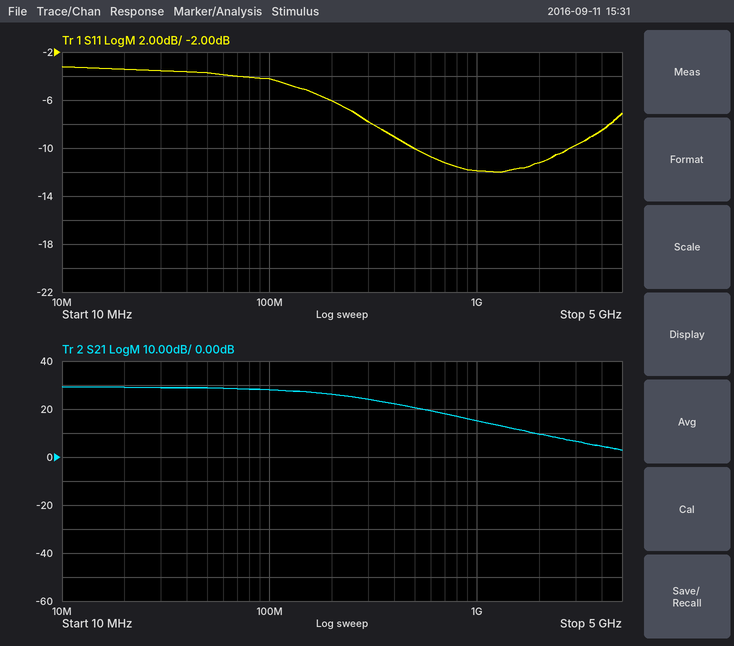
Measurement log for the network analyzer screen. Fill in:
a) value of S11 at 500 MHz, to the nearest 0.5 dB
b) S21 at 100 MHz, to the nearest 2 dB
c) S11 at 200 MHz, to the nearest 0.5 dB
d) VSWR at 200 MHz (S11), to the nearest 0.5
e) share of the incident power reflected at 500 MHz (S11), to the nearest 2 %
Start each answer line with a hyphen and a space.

- -10.0 dB
- 28 dB
- -6.0 dB
- 3.0
- 10 %
